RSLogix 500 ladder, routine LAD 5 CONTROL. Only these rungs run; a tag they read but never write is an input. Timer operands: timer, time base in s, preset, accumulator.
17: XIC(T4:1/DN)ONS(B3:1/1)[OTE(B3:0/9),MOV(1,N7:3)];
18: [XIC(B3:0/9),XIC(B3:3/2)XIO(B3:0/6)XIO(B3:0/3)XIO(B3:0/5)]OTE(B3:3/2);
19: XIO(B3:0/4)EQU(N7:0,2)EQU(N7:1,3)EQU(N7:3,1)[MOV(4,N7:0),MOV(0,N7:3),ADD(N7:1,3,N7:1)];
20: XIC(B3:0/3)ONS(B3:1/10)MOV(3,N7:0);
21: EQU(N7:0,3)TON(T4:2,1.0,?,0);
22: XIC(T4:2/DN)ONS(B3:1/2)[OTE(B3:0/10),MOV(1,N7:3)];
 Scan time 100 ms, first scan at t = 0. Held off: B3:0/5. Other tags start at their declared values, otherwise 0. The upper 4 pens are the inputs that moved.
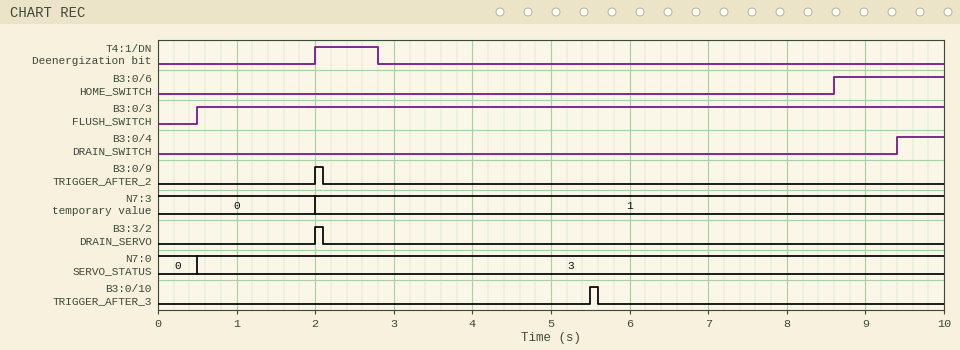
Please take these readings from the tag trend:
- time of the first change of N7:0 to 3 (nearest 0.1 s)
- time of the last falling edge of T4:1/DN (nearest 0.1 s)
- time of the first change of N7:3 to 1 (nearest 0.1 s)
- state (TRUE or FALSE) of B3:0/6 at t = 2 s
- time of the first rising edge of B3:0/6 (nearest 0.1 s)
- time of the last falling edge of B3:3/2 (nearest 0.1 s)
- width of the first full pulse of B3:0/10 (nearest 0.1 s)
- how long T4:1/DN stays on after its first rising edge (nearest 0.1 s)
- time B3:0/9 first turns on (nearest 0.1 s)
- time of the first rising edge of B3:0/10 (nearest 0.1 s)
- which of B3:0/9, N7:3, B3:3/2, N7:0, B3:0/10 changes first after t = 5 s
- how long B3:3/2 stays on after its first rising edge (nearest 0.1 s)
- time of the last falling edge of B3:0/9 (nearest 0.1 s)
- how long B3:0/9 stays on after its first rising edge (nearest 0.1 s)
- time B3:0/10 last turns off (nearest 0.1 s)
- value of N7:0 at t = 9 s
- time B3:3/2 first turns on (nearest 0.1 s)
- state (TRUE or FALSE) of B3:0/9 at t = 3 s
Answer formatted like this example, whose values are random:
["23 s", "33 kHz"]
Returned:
["0.5 s", "2.8 s", "2.0 s", "FALSE", "8.6 s", "2.1 s", "0.1 s", "0.8 s", "2.0 s", "5.5 s", "B3:0/10", "0.1 s", "2.1 s", "0.1 s", "5.6 s", "3", "2.0 s", "FALSE"]
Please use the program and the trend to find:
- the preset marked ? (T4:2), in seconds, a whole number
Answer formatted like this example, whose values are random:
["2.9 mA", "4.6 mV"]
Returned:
["5 s"]
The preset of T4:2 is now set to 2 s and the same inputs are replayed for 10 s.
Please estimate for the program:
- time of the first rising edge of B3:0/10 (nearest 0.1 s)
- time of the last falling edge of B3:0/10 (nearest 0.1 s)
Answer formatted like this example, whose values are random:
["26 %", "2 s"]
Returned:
["2.5 s", "2.6 s"]
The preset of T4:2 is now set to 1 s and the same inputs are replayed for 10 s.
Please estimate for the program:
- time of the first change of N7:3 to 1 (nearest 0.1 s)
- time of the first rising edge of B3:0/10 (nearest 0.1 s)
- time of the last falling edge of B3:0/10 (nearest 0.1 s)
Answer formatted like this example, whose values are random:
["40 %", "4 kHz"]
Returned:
["1.5 s", "1.5 s", "1.6 s"]
